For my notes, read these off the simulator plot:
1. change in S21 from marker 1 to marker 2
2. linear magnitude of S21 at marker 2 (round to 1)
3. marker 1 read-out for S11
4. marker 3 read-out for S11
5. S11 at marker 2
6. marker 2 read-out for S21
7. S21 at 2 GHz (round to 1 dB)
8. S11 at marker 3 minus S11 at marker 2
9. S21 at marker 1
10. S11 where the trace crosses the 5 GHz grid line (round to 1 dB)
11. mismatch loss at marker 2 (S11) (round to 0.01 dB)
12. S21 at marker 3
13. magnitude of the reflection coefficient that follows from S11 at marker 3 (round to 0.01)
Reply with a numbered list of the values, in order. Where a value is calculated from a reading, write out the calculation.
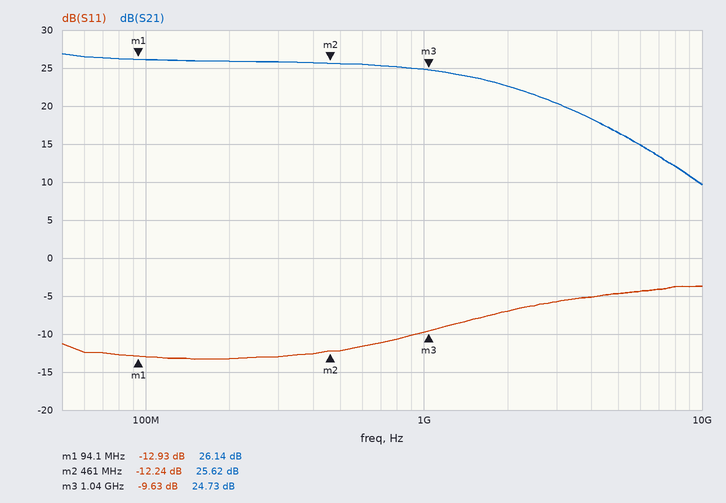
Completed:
1. 25.62 − (26.14) = -0.52 dB
2. 10^(25.62/20) ≈ 19
3. -12.93 dB
4. -9.63 dB
5. -12.24 dB
6. 25.62 dB
7. 23 dB
8. -9.63 − (-12.24) = 2.61 dB
9. 26.14 dB
10. -5 dB
11. −10 log10(1 − 10^(-12.24/10)) ≈ 0.27 dB
12. 24.73 dB
13. 10^(-9.63/20) ≈ 0.33
